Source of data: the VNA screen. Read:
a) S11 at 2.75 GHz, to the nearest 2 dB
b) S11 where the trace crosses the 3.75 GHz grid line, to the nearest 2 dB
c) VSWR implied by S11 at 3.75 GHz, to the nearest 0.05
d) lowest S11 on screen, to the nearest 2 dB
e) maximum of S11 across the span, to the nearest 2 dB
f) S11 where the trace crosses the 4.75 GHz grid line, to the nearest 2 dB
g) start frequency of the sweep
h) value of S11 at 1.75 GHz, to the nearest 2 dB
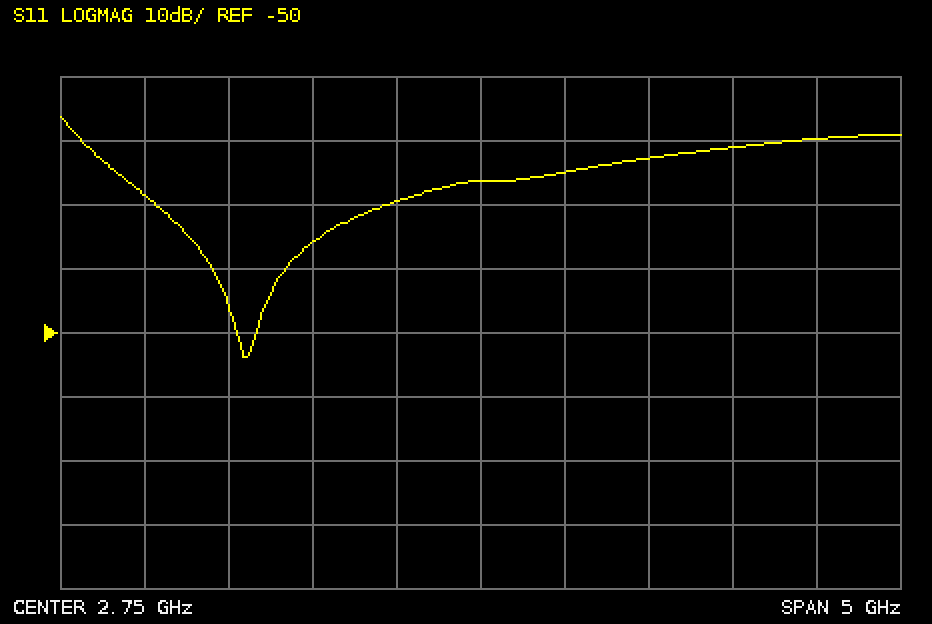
-26 dB
-22 dB
1.15
-54 dB
-16 dB
-20 dB
250 MHz
-36 dB
